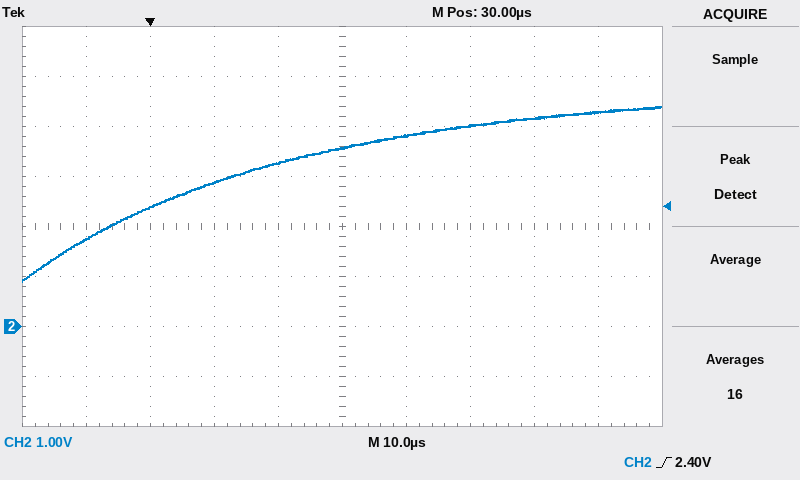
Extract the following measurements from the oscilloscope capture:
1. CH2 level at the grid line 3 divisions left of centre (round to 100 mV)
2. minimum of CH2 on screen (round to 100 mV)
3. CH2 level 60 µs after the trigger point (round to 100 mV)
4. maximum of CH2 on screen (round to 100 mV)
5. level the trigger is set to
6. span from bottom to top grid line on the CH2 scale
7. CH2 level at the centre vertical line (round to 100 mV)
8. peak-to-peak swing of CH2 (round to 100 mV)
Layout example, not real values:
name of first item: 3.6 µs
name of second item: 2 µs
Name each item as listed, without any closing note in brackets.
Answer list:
CH2 level at the grid line 3 divisions left of centre: 2.4 V
minimum of CH2 on screen: 900 mV
CH2 level 60 µs after the trigger point: 4.2 V
maximum of CH2 on screen: 4.4 V
level the trigger is set to: 2.40 V
span from bottom to top grid line on the CH2 scale: 8 V
CH2 level at the centre vertical line: 3.6 V
peak-to-peak swing of CH2: 3.5 V
